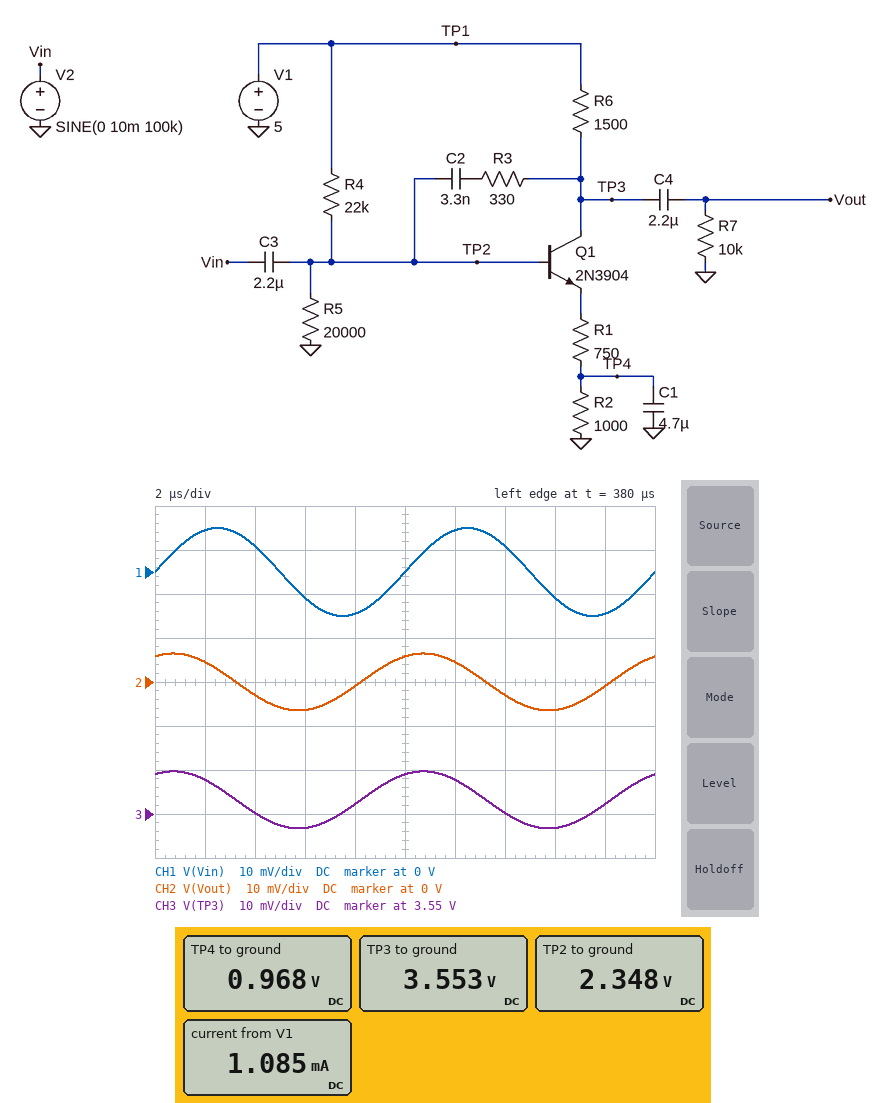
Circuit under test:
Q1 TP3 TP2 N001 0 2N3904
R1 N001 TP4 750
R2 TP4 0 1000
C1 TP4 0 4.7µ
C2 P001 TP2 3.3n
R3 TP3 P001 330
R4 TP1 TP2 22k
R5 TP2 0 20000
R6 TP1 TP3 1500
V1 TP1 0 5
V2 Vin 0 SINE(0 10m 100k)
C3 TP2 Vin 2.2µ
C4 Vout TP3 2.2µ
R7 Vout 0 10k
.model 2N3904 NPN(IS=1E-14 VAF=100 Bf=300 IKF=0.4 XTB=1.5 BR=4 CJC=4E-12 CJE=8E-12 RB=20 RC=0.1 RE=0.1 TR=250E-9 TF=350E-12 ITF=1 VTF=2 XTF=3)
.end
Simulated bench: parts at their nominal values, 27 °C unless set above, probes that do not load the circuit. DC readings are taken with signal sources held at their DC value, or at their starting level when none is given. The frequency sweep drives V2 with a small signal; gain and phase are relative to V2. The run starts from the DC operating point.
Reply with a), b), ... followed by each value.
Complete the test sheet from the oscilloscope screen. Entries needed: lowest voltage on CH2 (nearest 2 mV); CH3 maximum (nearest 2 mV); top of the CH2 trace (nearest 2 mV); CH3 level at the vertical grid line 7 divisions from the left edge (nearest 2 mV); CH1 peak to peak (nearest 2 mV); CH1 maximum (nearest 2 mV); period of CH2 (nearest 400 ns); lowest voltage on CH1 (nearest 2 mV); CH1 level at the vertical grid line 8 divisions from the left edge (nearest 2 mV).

a) -6 mV
b) 3.560 V
c) 6 mV
d) 3.550 V
e) 20 mV
f) 10 mV
g) 10.0 µs
h) -10 mV
i) -6 mV
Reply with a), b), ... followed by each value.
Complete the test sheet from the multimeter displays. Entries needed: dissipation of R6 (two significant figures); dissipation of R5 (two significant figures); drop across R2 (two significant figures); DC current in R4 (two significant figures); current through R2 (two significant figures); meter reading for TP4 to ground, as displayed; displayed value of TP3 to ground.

a) 1.4 mW
b) 280 µW
c) 970 mV
d) 120 µA
e) 970 µA
f) 0.968 V
g) 3.553 V
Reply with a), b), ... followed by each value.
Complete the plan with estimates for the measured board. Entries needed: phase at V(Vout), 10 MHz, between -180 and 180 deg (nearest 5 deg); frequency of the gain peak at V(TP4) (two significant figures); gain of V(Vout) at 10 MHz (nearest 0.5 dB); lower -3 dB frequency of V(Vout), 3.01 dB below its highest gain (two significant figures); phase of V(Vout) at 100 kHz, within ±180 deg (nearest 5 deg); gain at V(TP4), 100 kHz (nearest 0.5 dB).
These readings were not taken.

a) 5 deg
b) 23 Hz
c) -6.5 dB
d) 62 Hz
e) 65 deg
f) -67.0 dB
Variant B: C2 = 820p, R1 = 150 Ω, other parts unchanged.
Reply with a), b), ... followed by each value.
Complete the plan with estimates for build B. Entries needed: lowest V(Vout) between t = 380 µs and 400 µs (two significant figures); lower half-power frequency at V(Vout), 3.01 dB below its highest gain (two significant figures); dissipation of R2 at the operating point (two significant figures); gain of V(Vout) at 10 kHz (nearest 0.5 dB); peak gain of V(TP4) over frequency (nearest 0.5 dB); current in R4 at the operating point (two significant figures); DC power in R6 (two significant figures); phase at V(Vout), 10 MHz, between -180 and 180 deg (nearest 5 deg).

a) -59 mV
b) 230 Hz
c) 2.1 mW
d) 17.5 dB
e) -1.5 dB
f) 120 µA
g) 3.1 mW
h) 160 deg
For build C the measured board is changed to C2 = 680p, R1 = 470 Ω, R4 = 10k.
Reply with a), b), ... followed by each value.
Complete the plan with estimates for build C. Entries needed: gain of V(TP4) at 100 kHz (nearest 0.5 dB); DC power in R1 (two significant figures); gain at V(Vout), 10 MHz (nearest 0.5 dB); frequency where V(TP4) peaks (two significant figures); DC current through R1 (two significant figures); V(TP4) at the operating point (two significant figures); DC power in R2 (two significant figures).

a) -64.0 dB
b) 1.3 mW
c) -0.5 dB
d) 81 Hz
e) 1.7 mA
f) 1.7 V
g) 2.8 mW
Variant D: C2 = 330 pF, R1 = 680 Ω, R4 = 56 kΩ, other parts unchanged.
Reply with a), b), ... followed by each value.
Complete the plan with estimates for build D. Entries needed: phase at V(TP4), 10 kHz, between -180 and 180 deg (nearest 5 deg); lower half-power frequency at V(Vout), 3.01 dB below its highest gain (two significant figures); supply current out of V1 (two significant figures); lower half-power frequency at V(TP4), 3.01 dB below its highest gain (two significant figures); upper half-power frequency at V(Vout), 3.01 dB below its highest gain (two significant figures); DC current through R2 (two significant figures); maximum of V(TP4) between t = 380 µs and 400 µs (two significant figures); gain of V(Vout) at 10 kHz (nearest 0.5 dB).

a) -90 deg
b) 65 Hz
c) 460 µA
d) 4.5 Hz
e) 320 kHz
f) 400 µA
g) 400 mV
h) 5.0 dB
